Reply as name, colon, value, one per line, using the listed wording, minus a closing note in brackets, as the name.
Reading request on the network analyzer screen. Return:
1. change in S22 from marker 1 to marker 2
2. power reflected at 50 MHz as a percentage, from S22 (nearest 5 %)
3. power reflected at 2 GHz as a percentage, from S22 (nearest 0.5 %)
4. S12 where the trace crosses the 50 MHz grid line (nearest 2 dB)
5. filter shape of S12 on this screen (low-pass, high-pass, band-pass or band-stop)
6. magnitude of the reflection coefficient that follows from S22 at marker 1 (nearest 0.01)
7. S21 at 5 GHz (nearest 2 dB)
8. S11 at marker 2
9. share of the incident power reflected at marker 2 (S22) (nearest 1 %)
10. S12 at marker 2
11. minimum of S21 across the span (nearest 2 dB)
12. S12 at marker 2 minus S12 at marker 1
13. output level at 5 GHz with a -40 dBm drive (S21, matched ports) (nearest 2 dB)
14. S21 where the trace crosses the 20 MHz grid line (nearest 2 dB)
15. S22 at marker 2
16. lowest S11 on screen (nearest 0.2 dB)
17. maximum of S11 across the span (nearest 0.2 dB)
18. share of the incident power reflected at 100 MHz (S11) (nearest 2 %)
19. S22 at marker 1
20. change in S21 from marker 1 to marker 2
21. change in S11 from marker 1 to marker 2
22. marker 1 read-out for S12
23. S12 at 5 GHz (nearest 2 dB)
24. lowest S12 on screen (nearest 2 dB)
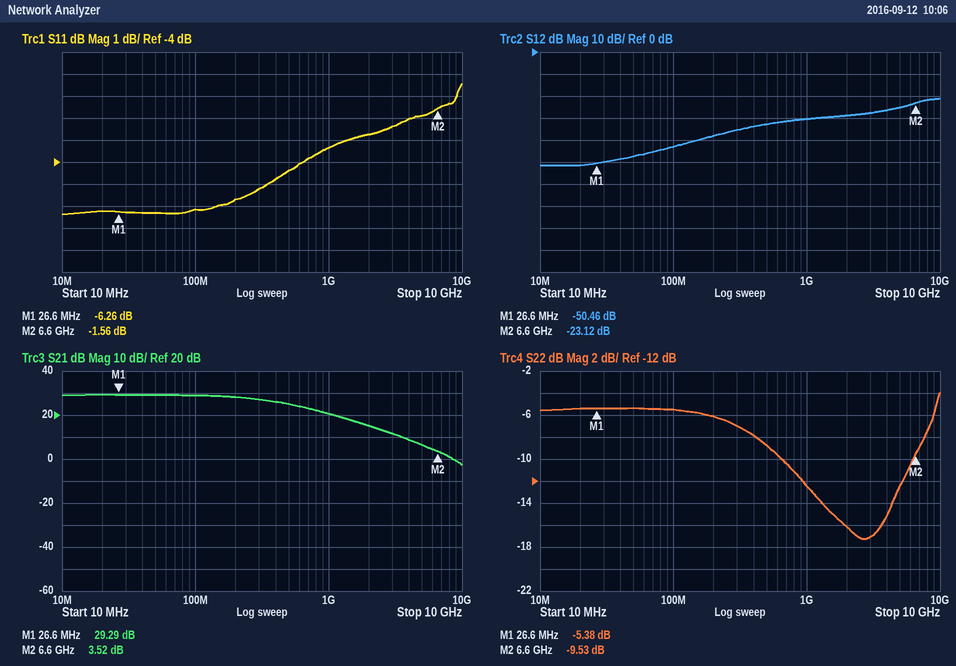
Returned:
change in S22 from marker 1 to marker 2: -4.15 dB
power reflected at 50 MHz as a percentage, from S22: 30 %
power reflected at 2 GHz as a percentage, from S22: 2.5 %
S12 where the trace crosses the 50 MHz grid line: -48 dB
filter shape of S12 on this screen: high-pass
magnitude of the reflection coefficient that follows from S22 at marker 1: 0.54
S21 at 5 GHz: 6 dB
S11 at marker 2: -1.56 dB
share of the incident power reflected at marker 2 (S22): 11 %
S12 at marker 2: -23.12 dB
minimum of S21 across the span: -2 dB
S12 at marker 2 minus S12 at marker 1: 27.34 dB
output level at 5 GHz with a -40 dBm drive (S21, matched ports): -34 dBm
S21 where the trace crosses the 20 MHz grid line: 30 dB
S22 at marker 2: -9.53 dB
lowest S11 on screen: -6.4 dB
maximum of S11 across the span: -0.4 dB
share of the incident power reflected at 100 MHz (S11): 24 %
S22 at marker 1: -5.38 dB
change in S21 from marker 1 to marker 2: -25.77 dB
change in S11 from marker 1 to marker 2: 4.70 dB
marker 1 read-out for S12: -50.46 dB
S12 at 5 GHz: -26 dB
lowest S12 on screen: -52 dB
